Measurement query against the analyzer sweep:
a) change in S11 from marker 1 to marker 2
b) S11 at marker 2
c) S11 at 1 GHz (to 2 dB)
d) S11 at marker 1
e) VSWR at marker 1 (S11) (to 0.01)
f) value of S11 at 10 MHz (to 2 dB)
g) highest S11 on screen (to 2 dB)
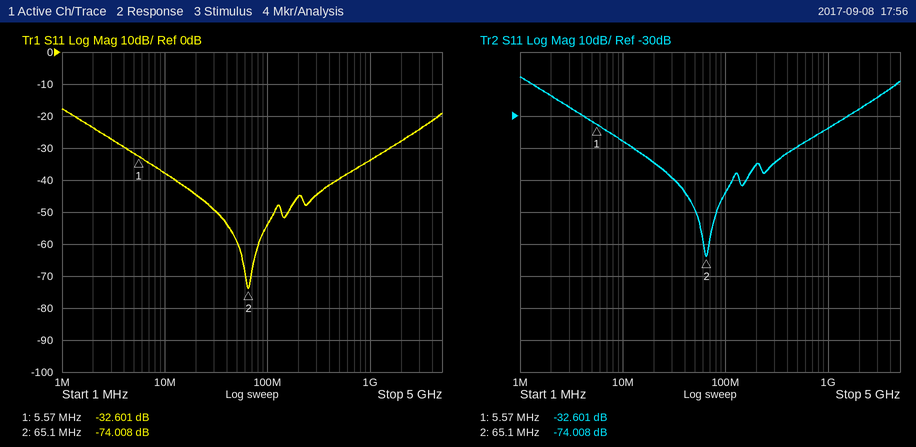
-41.407 dB
-74.008 dB
-34 dB
-32.601 dB
1.05
-38 dB
-18 dB
